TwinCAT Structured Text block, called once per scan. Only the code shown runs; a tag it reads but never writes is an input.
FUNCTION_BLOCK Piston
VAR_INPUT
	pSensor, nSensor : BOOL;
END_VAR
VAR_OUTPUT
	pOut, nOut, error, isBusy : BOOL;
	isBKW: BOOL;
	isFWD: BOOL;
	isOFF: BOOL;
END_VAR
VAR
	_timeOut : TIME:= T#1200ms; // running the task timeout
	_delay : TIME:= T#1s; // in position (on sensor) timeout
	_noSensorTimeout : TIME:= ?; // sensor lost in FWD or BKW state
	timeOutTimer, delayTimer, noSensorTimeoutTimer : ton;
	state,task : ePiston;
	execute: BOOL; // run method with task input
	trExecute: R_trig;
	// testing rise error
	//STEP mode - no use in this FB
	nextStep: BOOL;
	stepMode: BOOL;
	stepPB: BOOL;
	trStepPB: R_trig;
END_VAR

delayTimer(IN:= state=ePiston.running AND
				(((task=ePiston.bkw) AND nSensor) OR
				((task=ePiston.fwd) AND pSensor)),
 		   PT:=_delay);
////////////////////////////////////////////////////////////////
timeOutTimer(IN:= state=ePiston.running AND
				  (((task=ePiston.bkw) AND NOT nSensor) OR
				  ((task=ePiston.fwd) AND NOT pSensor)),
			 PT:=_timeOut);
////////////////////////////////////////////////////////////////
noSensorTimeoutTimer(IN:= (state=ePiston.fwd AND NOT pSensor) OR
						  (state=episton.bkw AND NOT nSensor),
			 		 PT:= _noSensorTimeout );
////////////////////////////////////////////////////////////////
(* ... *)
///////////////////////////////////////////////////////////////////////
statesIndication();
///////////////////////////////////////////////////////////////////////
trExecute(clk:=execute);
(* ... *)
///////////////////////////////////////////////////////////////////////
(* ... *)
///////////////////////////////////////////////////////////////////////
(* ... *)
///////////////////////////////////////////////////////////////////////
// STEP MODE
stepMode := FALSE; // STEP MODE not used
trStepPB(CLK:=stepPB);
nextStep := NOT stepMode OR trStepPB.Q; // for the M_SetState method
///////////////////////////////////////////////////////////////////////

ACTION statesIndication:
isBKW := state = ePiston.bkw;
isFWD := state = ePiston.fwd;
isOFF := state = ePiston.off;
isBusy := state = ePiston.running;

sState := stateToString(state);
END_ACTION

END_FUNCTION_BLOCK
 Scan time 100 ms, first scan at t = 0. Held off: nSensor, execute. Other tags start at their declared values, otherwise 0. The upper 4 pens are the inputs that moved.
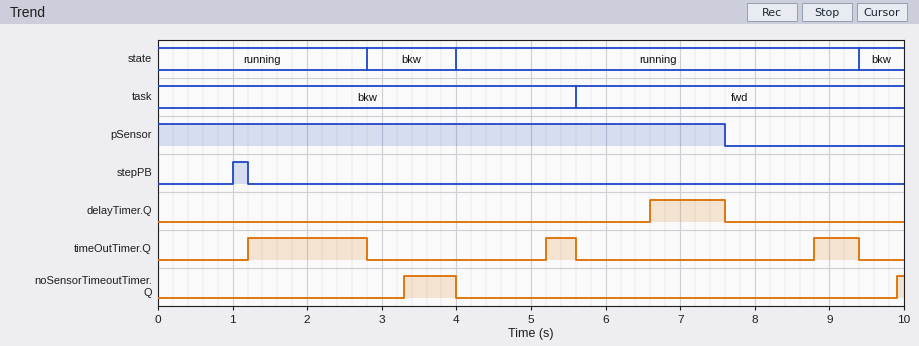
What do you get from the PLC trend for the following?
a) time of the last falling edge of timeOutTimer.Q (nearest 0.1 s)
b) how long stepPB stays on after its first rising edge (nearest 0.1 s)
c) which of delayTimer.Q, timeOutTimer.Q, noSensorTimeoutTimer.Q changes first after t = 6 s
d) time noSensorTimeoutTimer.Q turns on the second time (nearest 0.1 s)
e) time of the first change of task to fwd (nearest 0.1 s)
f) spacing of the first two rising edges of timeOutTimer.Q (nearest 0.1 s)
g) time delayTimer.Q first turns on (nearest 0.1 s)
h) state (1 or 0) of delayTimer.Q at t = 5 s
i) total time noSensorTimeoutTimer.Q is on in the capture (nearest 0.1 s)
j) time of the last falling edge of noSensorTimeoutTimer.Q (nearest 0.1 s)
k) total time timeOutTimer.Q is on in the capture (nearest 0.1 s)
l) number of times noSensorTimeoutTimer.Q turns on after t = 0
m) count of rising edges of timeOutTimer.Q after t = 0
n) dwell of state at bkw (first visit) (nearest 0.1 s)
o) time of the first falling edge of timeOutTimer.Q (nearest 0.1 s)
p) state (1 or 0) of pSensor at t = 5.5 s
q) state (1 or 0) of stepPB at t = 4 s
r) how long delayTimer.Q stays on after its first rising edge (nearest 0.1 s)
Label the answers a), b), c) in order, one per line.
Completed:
a) 9.4 s
b) 0.2 s
c) delayTimer.Q
d) 9.9 s
e) 5.6 s
f) 4.0 s
g) 6.6 s
h) 0
i) 0.8 s
j) 4.0 s
k) 2.6 s
l) 2
m) 3
n) 1.2 s
o) 2.8 s
p) 1
q) 0
r) 1.0 s
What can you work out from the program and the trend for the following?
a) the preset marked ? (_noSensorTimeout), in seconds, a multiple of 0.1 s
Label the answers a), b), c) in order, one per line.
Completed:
a) 0.5 s
